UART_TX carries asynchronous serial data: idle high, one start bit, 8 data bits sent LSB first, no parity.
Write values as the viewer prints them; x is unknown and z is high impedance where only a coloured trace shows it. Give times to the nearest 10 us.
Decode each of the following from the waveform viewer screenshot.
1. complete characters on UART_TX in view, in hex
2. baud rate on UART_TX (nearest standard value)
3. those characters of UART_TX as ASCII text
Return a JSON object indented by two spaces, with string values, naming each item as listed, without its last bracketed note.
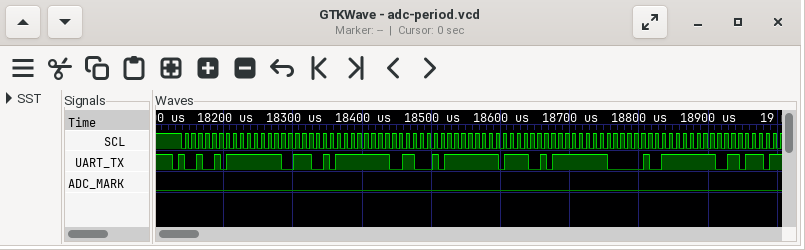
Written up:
{
  "complete characters on UART_TX in view, in hex": "49, 4E, 46, 4F, 20, 76",
  "baud rate on UART_TX": "115200 baud",
  "those characters of UART_TX as ASCII text": "\"INFO v\""
}
